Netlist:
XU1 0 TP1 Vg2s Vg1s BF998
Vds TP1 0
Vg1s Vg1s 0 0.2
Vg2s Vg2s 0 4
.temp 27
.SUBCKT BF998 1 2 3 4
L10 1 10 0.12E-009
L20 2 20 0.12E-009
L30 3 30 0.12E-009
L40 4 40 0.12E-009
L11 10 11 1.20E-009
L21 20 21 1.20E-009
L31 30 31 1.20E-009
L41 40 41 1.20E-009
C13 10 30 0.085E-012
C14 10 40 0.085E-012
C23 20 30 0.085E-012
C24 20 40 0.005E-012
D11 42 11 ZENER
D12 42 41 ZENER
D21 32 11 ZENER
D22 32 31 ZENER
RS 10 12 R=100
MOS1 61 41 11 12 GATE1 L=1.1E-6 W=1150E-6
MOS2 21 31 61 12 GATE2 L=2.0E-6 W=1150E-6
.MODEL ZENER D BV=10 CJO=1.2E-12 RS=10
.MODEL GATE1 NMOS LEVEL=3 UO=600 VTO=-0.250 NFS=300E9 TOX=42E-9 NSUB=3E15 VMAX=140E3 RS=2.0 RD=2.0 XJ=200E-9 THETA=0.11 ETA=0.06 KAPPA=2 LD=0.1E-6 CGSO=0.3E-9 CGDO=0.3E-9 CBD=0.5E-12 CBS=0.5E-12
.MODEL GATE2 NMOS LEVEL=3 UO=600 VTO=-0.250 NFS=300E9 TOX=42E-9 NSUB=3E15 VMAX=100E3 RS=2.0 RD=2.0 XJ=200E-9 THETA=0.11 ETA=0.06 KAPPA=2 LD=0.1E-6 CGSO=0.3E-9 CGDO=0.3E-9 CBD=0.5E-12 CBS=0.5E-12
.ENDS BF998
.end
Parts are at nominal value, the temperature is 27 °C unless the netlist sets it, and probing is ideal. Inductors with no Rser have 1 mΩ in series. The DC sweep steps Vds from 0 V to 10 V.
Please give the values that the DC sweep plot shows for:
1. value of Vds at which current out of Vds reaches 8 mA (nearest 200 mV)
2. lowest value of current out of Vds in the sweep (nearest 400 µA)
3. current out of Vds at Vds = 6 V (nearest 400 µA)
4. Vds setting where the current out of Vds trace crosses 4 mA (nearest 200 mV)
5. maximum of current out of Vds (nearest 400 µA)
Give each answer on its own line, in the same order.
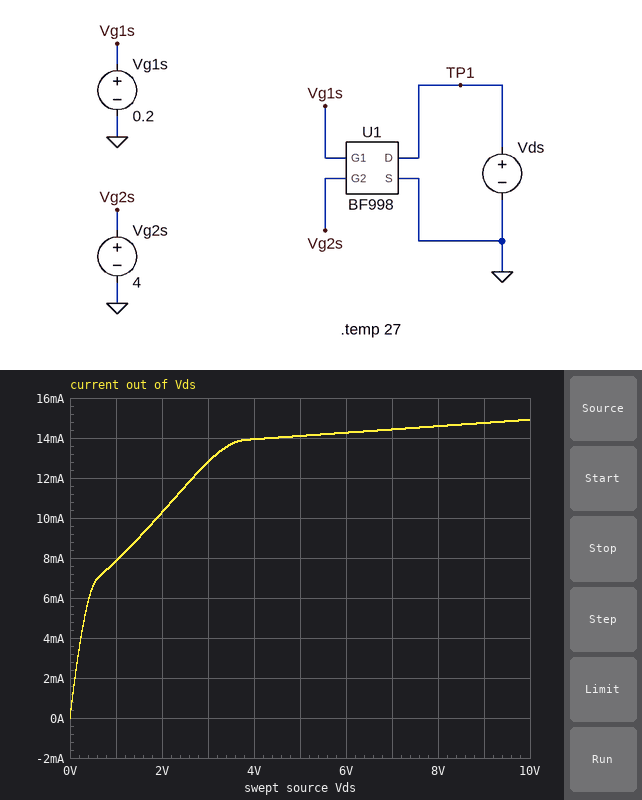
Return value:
1.0 V
0 A
14.4 mA
200 mV
14.8 mA
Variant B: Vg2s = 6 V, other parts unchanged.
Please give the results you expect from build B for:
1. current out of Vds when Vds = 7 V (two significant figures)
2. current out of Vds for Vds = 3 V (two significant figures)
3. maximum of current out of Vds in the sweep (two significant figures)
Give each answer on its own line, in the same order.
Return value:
22 mA
14 mA
23 mA
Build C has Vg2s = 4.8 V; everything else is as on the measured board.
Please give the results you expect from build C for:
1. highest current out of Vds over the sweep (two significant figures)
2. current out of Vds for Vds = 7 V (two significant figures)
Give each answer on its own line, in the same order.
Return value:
18 mA
17 mA
